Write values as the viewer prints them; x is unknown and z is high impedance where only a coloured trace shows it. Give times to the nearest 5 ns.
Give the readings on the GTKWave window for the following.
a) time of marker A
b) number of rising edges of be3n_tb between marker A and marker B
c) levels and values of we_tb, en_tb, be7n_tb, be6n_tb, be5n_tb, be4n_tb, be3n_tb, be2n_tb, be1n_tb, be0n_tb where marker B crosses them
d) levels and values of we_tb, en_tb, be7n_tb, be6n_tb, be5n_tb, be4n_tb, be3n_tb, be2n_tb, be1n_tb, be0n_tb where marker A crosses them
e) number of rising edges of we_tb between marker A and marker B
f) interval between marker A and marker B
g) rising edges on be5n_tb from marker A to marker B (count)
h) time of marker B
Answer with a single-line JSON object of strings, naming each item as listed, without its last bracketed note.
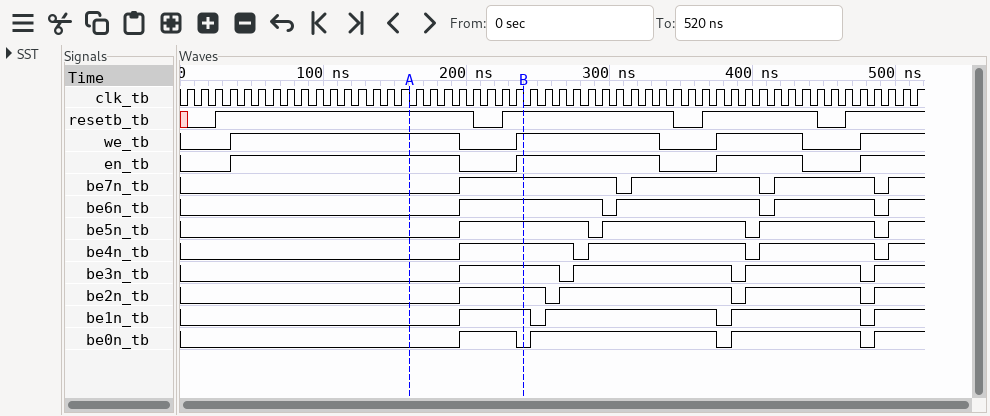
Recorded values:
{"time of marker A": "160 ns", "number of rising edges of be3n_tb between marker A and marker B": "1", "levels and values of we_tb, en_tb, be7n_tb, be6n_tb, be5n_tb, be4n_tb, be3n_tb, be2n_tb, be1n_tb, be0n_tb where marker B crosses them": "we_tb=1, en_tb=1, be7n_tb=1, be6n_tb=1, be5n_tb=1, be4n_tb=1, be3n_tb=1, be2n_tb=1, be1n_tb=1, be0n_tb=0", "levels and values of we_tb, en_tb, be7n_tb, be6n_tb, be5n_tb, be4n_tb, be3n_tb, be2n_tb, be1n_tb, be0n_tb where marker A crosses them": "we_tb=1, en_tb=1, be7n_tb=0, be6n_tb=0, be5n_tb=0, be4n_tb=0, be3n_tb=0, be2n_tb=0, be1n_tb=0, be0n_tb=0", "number of rising edges of we_tb between marker A and marker B": "1", "interval between marker A and marker B": "80 ns", "rising edges on be5n_tb from marker A to marker B": "1", "time of marker B": "240 ns"}
